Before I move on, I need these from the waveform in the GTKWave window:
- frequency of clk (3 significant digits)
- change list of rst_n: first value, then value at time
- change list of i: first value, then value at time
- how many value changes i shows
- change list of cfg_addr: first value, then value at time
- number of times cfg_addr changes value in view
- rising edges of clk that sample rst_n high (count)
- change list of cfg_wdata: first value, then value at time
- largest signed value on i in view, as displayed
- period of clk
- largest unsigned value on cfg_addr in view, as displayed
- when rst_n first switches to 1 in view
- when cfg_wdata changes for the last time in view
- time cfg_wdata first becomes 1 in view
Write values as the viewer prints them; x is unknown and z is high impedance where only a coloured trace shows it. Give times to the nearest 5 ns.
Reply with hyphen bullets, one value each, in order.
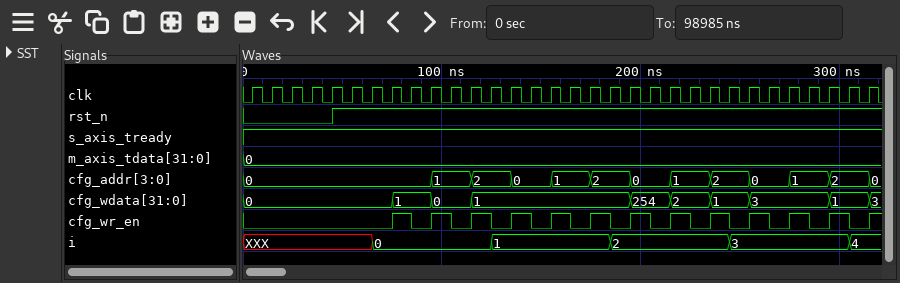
- 100 MHz
- 0, 1 at 45 ns
- XXX, 0 at 65 ns, 1 at 125 ns, 2 at 185 ns, 3 at 245 ns, 4 at 305 ns
- 5
- 0, 1 at 95 ns, 2 at 115 ns, 0 at 135 ns, 1 at 155 ns, 2 at 175 ns, 0 at 195 ns, 1 at 215 ns, 2 at 235 ns, 0 at 255 ns, 1 at 275 ns, 2 at 295 ns, 0 at 315 ns
- 12
- 27
- 0, 1 at 75 ns, 0 at 95 ns, 1 at 115 ns, 254 at 195 ns, 2 at 215 ns, 1 at 235 ns, 3 at 255 ns, 1 at 295 ns, 3 at 315 ns
- 4
- 10 ns
- 2
- 45 ns
- 315 ns
- 75 ns
